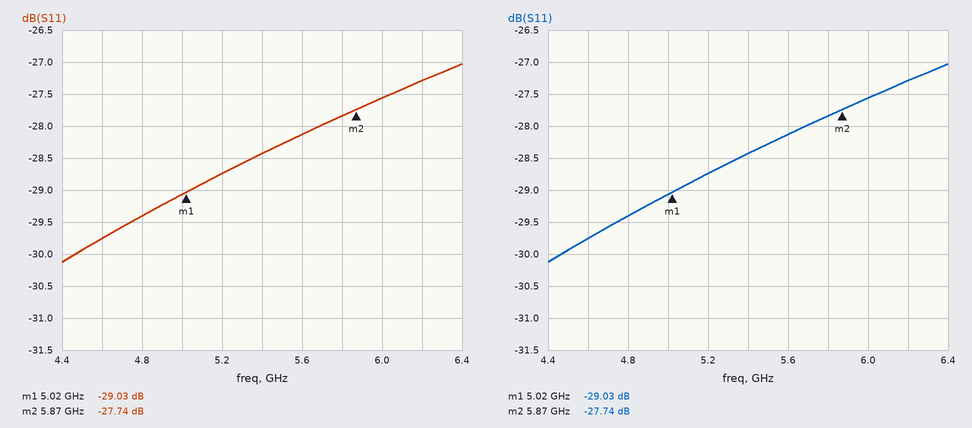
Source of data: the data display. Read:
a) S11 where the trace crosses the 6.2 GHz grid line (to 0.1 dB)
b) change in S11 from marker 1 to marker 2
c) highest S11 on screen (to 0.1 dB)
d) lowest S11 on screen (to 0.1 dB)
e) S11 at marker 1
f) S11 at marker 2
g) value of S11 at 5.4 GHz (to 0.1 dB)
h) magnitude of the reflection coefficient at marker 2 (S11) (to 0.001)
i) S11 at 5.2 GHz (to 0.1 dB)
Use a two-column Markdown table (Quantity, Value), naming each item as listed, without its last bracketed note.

| Quantity | Value |
|---|---|
| S11 where the trace crosses the 6.2 GHz grid line | -27.3 dB |
| change in S11 from marker 1 to marker 2 | 1.29 dB |
| highest S11 on screen | -27.0 dB |
| lowest S11 on screen | -30.1 dB |
| S11 at marker 1 | -29.03 dB |
| S11 at marker 2 | -27.74 dB |
| value of S11 at 5.4 GHz | -28.4 dB |
| magnitude of the reflection coefficient at marker 2 (S11) | 0.041 |
| S11 at 5.2 GHz | -28.7 dB |
